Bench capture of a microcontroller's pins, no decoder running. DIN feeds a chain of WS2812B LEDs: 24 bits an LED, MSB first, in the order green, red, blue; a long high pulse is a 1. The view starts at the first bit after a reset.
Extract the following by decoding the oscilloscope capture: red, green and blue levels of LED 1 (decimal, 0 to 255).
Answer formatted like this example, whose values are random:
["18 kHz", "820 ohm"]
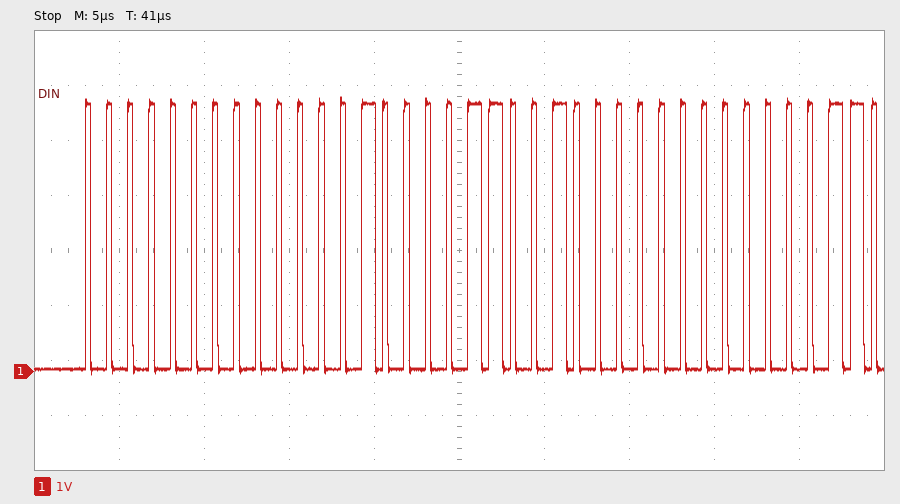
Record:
["4, 0, 50"]
